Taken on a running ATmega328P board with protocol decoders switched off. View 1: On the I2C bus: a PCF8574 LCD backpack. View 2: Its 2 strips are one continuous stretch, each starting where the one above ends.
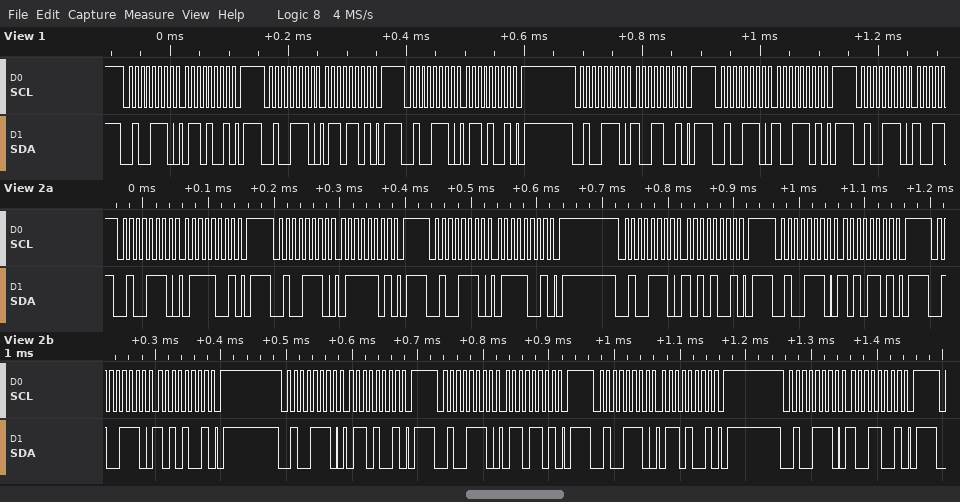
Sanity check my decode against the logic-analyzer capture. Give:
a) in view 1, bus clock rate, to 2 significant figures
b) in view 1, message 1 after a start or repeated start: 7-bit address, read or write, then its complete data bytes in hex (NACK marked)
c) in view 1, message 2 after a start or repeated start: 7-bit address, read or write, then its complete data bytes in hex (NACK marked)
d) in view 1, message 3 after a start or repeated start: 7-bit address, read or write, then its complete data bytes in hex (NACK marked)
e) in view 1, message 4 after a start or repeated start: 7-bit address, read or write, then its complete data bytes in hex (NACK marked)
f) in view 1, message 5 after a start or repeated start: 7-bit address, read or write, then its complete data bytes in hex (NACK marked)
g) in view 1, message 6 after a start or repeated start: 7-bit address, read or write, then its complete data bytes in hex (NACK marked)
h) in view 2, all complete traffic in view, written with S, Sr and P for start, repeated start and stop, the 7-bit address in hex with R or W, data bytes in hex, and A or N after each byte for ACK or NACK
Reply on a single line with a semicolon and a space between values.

100 kHz; 0x27 write: 69; 0x27 write: 6D; 0x27 write: 69; 0x27 write: 99; 0x27 write: 9D; 0x27 write; S 27W A 79 A P S 27W A 7D A P S 27W A 79 A P S 27W A A9 A P S 27W A AD A P S 27W A A9 A P S 27W A 69 A P S 27W A 6D A P S 27W A 69 A P S 27W A 99 A P
